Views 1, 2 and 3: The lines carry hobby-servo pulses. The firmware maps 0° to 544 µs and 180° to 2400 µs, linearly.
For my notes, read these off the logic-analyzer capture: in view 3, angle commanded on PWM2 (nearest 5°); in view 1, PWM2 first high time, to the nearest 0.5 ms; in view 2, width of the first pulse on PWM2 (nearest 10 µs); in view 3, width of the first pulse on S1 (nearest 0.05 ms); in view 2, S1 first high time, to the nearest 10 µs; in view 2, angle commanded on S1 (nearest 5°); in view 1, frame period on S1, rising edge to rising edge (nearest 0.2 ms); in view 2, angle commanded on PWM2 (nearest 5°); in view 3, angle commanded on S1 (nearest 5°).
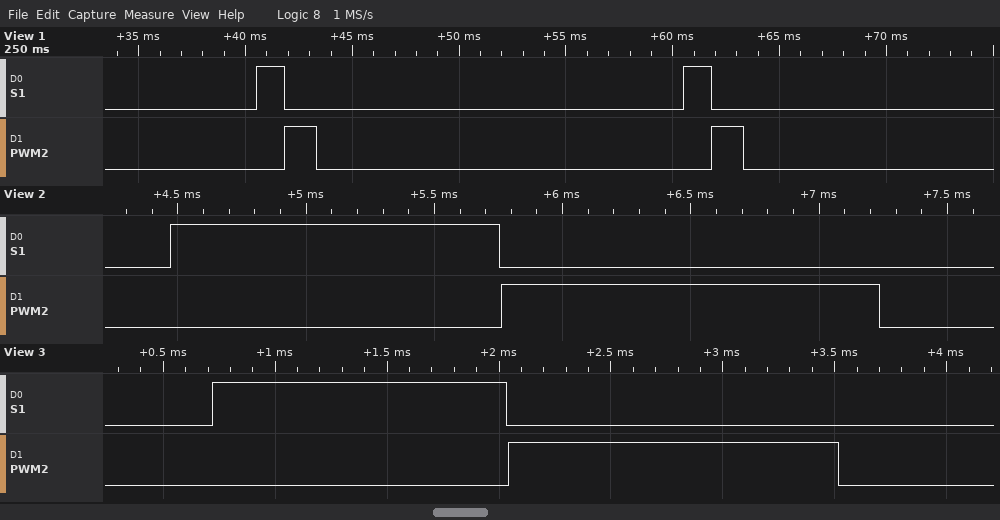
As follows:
90°
1.5 ms
1470 µs
1.30 ms
1280 µs
70°
20.0 ms
90°
75°
